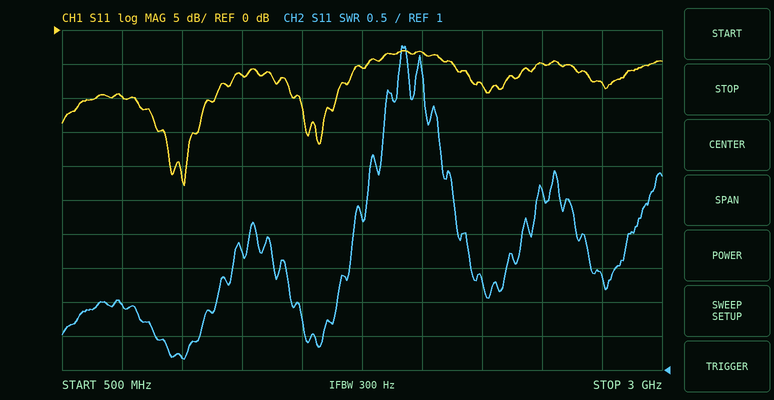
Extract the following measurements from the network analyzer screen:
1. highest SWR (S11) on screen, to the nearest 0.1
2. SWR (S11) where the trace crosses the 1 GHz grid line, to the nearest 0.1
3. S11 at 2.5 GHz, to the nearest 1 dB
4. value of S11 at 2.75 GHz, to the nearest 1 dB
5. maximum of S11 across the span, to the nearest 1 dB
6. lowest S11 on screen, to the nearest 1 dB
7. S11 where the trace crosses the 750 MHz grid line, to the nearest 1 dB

5.8
1.2
-5 dB
-8 dB
-3 dB
-23 dB
-10 dB
